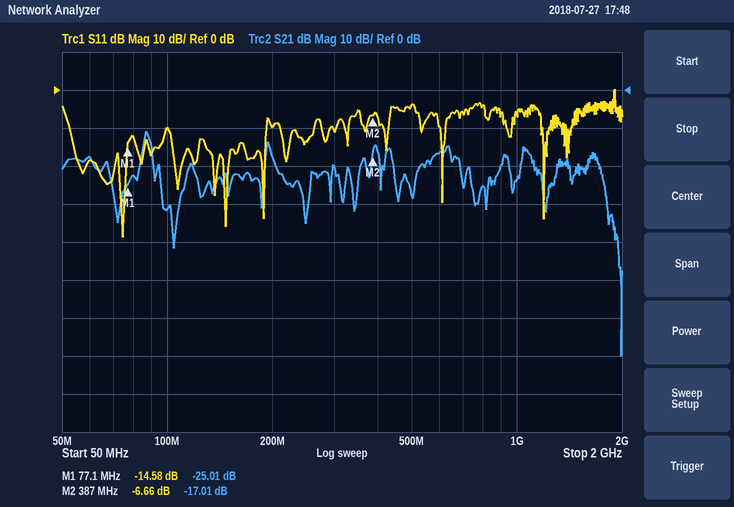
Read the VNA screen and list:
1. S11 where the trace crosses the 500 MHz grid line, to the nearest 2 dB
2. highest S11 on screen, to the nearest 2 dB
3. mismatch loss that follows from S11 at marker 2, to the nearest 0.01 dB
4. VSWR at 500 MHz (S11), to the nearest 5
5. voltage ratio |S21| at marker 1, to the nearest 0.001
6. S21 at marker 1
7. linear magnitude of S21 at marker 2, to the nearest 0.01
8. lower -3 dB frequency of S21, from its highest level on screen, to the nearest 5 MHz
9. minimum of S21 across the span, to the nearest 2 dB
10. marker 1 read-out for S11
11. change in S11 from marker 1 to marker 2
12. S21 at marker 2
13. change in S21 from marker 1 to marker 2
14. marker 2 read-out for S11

-4 dB
0 dB
1.06 dB
5
0.056
-25.01 dB
0.14
85 MHz
-70 dB
-14.58 dB
7.92 dB
-17.01 dB
8.00 dB
-6.66 dB
